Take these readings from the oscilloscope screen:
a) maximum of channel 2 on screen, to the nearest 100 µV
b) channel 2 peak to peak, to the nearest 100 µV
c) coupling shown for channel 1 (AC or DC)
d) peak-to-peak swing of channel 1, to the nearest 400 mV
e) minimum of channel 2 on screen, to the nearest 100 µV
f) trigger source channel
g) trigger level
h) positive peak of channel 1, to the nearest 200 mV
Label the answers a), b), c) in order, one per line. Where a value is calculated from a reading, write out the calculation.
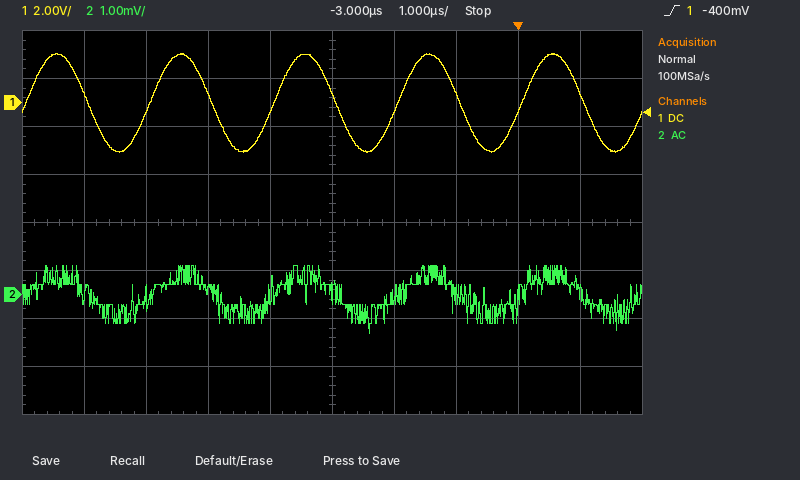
a) 600 µV
b) 600 µV − (-800 µV) = 1.4 mV
c) DC
d) 4.0 V
e) -800 µV
f) channel 1
g) -400 mV
h) 2.0 V
